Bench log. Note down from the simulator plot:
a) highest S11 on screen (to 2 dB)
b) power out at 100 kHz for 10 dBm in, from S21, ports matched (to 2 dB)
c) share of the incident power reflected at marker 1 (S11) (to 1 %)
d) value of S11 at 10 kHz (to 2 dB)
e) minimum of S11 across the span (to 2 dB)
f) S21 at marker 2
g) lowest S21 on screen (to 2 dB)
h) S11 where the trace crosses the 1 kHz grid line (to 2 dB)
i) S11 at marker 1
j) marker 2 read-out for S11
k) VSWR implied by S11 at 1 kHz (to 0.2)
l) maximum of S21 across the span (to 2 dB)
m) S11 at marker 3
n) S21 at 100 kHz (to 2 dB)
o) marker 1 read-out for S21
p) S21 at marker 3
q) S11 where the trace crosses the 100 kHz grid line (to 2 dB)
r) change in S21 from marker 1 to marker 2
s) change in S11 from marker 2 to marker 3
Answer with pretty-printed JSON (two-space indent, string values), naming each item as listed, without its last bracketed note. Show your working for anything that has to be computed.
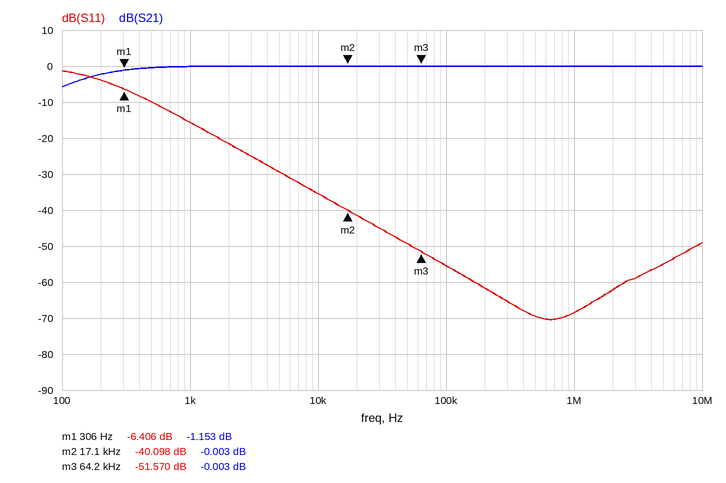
{
  "highest S11 on screen": "-2 dB",
  "power out at 100 kHz for 10 dBm in, from S21, ports matched": "10 dBm + (0 dB) = 10 dBm",
  "share of the incident power reflected at marker 1 (S11)": "10^(-6.406/10) ≈ 23 %",
  "value of S11 at 10 kHz": "-36 dB",
  "minimum of S11 across the span": "-70 dB",
  "S21 at marker 2": "-0.003 dB",
  "lowest S21 on screen": "-6 dB",
  "S11 where the trace crosses the 1 kHz grid line": "-16 dB",
  "S11 at marker 1": "-6.406 dB",
  "marker 2 read-out for S11": "-40.098 dB",
  "VSWR implied by S11 at 1 kHz": "|Γ| = 10^(-16/20) = 0.1585; VSWR = (1 + 0.1585)/(1 − 0.1585) ≈ 1.4",
  "maximum of S21 across the span": "0 dB",
  "S11 at marker 3": "-51.570 dB",
  "S21 at 100 kHz": "0 dB",
  "marker 1 read-out for S21": "-1.153 dB",
  "S21 at marker 3": "-0.003 dB",
  "S11 where the trace crosses the 100 kHz grid line": "-56 dB",
  "change in S21 from marker 1 to marker 2": "-0.003 − (-1.153) = 1.150 dB",
  "change in S11 from marker 2 to marker 3": "-51.57 − (-40.098) = -11.472 dB"
}
